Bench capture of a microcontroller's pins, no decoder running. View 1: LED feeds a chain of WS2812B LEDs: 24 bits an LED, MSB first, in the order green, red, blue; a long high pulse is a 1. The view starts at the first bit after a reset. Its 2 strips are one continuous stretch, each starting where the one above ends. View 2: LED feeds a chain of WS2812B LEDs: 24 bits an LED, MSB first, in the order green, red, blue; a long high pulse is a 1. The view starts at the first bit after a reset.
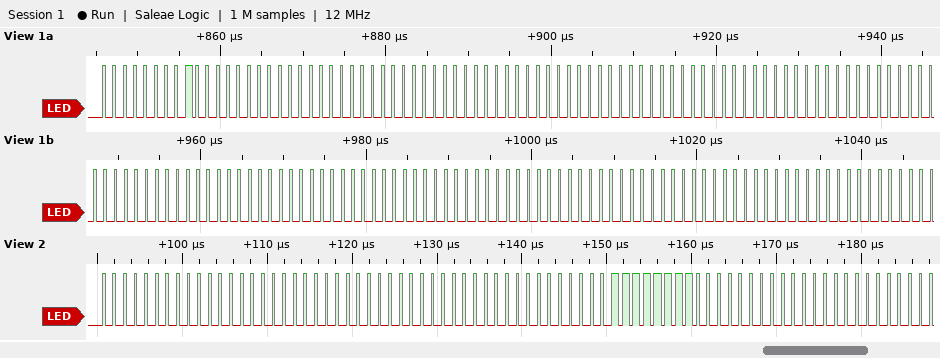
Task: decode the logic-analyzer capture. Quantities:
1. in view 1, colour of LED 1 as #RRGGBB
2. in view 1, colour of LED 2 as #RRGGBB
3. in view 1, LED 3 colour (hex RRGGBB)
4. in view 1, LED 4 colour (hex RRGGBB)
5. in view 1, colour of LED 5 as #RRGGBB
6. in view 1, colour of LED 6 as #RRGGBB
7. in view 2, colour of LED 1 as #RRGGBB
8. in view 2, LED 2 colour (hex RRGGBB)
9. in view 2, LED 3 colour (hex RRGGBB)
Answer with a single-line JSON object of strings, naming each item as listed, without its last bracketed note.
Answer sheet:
{"in view 1, colour of LED 1 as #RRGGBB": "#800000", "in view 1, colour of LED 2 as #RRGGBB": "#000000", "in view 1, LED 3 colour": "#000000", "in view 1, LED 4 colour": "#000000", "in view 1, colour of LED 5 as #RRGGBB": "#000000", "in view 1, colour of LED 6 as #RRGGBB": "#000000", "in view 2, colour of LED 1 as #RRGGBB": "#000000", "in view 2, LED 2 colour": "#000000", "in view 2, LED 3 colour": "#00FF00"}
